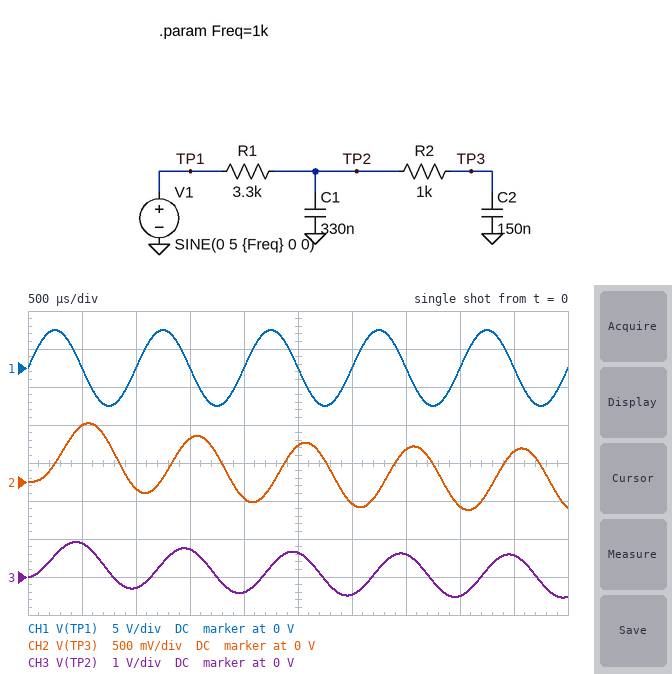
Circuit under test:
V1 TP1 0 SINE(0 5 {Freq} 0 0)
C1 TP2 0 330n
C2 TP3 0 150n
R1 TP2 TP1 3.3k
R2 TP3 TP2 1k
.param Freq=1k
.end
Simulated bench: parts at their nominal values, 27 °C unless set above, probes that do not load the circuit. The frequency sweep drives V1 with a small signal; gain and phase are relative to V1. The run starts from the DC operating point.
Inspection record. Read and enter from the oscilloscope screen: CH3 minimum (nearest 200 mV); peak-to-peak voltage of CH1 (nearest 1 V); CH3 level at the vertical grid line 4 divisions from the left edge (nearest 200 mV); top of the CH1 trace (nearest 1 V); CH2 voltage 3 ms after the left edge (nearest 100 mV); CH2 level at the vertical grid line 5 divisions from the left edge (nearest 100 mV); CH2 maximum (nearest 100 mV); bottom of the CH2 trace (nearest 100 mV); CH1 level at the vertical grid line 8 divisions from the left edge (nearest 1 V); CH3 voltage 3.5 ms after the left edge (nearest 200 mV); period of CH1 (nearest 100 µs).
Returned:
-600 mV
10 V
-400 mV
5 V
-300 mV
500 mV
800 mV
-400 mV
0 V
600 mV
1.0 ms
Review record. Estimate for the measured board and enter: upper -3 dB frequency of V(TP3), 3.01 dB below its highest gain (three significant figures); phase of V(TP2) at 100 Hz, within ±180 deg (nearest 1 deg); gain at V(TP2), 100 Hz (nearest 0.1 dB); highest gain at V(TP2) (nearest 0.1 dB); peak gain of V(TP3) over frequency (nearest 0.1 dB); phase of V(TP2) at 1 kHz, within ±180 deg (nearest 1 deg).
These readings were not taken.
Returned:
97.0 Hz
-44 deg
-3.1 dB
0 dB
0 dB
-73 deg
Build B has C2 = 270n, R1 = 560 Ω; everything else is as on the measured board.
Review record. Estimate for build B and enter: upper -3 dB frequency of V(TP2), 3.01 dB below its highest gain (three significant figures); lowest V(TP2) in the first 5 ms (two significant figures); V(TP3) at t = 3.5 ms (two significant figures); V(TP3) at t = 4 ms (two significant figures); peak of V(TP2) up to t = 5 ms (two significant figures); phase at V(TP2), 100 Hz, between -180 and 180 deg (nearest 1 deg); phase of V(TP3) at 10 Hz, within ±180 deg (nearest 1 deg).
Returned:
426 Hz
-2.5 V
1.2 V
-1.2 V
2.9 V
-12 deg
-2 deg
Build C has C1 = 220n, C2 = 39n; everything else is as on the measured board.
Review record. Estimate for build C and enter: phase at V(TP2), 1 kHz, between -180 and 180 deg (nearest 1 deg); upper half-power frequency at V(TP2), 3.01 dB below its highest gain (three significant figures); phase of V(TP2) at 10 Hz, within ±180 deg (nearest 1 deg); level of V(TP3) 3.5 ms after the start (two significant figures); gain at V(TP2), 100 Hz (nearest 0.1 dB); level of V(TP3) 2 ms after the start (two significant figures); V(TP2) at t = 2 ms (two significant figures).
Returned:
-77 deg
185 Hz
-3 deg
910 mV
-1.1 dB
-800 mV
-810 mV
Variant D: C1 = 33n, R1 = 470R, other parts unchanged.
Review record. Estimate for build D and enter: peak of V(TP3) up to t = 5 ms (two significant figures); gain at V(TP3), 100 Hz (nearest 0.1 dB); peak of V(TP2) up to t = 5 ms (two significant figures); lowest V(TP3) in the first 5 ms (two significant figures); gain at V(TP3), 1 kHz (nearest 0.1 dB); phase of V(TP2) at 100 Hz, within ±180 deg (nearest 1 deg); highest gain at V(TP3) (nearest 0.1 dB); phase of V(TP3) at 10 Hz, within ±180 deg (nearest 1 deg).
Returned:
3.3 V
-0.1 dB
4.2 V
-2.9 V
-4.8 dB
-3 deg
0 dB
-1 deg
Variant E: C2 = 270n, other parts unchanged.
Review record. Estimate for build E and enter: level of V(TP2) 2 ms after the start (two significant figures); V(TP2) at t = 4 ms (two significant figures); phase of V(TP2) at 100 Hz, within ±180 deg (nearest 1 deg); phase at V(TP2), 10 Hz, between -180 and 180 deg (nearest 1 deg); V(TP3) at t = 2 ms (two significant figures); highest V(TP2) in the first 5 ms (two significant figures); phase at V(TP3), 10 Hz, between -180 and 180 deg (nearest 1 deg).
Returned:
-380 mV
-460 mV
-48 deg
-7 deg
-71 mV
850 mV
-8 deg
